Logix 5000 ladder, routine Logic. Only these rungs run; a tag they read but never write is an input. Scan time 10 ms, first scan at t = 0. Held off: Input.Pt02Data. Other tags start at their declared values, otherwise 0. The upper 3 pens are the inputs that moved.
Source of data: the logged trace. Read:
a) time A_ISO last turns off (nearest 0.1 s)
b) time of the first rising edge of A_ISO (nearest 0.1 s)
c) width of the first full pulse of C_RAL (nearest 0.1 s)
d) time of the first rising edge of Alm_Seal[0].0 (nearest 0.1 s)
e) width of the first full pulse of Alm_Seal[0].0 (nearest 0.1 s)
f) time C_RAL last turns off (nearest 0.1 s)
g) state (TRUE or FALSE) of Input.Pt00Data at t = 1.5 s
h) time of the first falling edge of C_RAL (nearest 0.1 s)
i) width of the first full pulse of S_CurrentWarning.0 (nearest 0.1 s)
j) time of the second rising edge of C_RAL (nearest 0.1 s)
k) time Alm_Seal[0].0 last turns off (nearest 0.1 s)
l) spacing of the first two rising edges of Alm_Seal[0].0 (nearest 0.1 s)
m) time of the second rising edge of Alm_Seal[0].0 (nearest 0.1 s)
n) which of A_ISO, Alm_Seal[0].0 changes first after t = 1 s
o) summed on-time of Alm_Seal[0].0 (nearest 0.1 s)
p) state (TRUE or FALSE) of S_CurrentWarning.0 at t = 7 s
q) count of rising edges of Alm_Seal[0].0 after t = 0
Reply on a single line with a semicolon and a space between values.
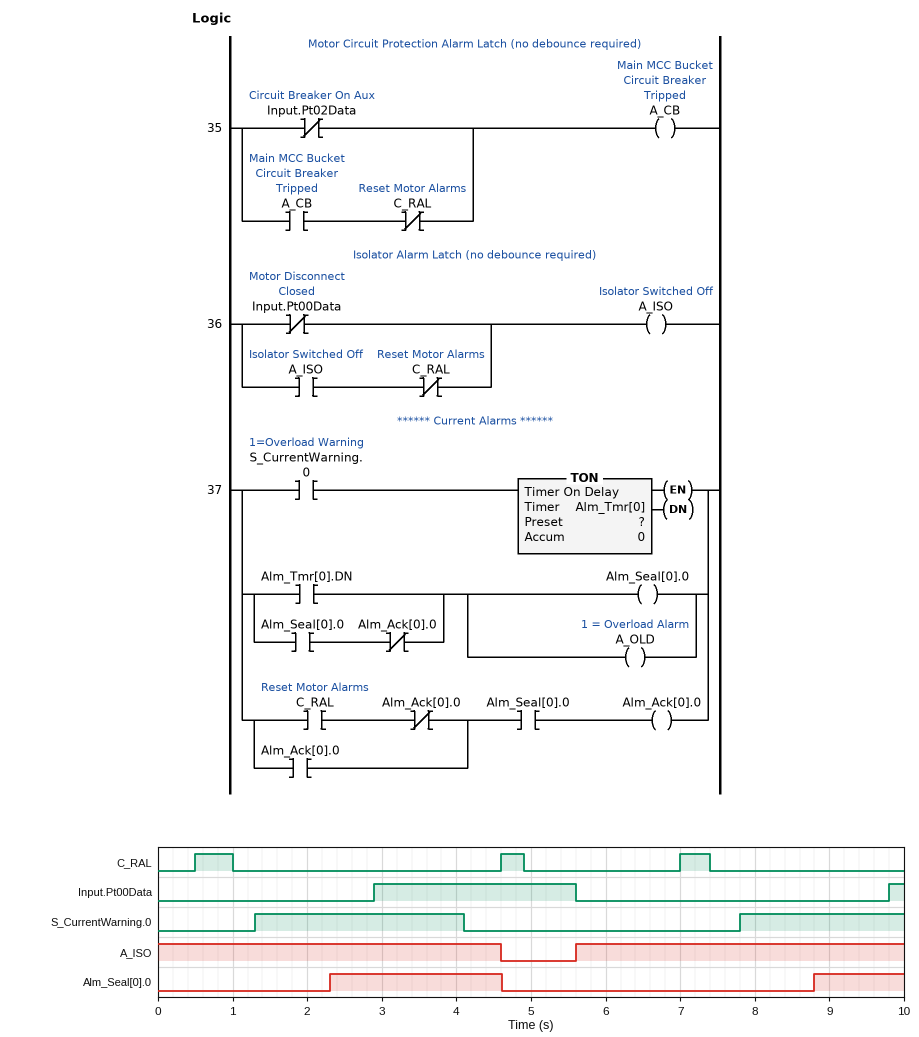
4.6 s; 5.6 s; 0.5 s; 2.3 s; 2.3 s; 7.4 s; FALSE; 1.0 s; 2.8 s; 4.6 s; 4.6 s; 6.5 s; 8.8 s; Alm_Seal[0].0; 3.5 s; FALSE; 2
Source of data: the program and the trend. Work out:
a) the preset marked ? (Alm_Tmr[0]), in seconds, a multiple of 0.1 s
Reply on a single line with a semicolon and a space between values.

1.0 s
